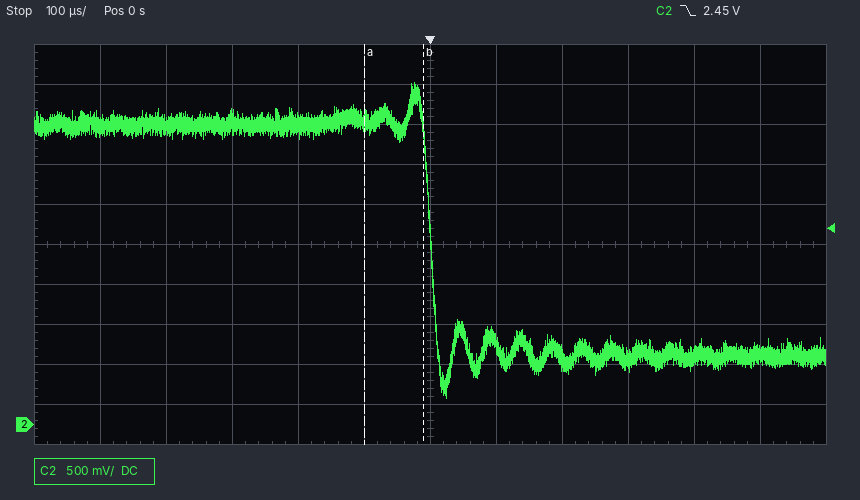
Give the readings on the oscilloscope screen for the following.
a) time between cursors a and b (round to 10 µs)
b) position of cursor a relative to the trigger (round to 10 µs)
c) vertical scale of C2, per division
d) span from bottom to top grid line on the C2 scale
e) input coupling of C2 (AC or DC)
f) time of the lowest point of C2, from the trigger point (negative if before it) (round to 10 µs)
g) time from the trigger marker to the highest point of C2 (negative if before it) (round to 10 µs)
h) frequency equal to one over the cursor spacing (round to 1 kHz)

90 µs
-100 µs
500 mV
5 V
DC
+20 µs
-20 µs
11 kHz
